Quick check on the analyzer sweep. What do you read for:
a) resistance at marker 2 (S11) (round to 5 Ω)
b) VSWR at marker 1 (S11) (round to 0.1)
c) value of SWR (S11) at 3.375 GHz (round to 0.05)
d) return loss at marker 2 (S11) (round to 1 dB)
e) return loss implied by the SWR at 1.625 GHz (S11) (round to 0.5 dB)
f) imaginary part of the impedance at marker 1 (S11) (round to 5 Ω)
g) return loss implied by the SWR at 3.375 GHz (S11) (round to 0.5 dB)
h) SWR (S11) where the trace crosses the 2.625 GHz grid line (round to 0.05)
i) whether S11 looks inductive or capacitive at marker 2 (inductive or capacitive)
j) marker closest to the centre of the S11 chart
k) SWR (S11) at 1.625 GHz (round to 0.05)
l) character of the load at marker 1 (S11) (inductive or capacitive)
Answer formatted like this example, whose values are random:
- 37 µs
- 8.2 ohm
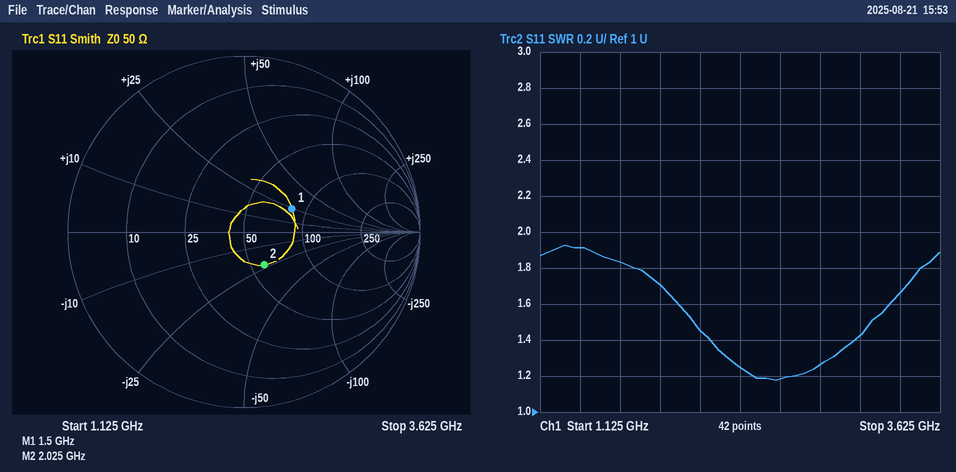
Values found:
- 60 Ω
- 1.9
- 1.65
- 13 dB
- 10.5 dB
- +25 Ω
- 12.0 dB
- 1.20
- capacitive
- marker 2
- 1.85
- inductive
